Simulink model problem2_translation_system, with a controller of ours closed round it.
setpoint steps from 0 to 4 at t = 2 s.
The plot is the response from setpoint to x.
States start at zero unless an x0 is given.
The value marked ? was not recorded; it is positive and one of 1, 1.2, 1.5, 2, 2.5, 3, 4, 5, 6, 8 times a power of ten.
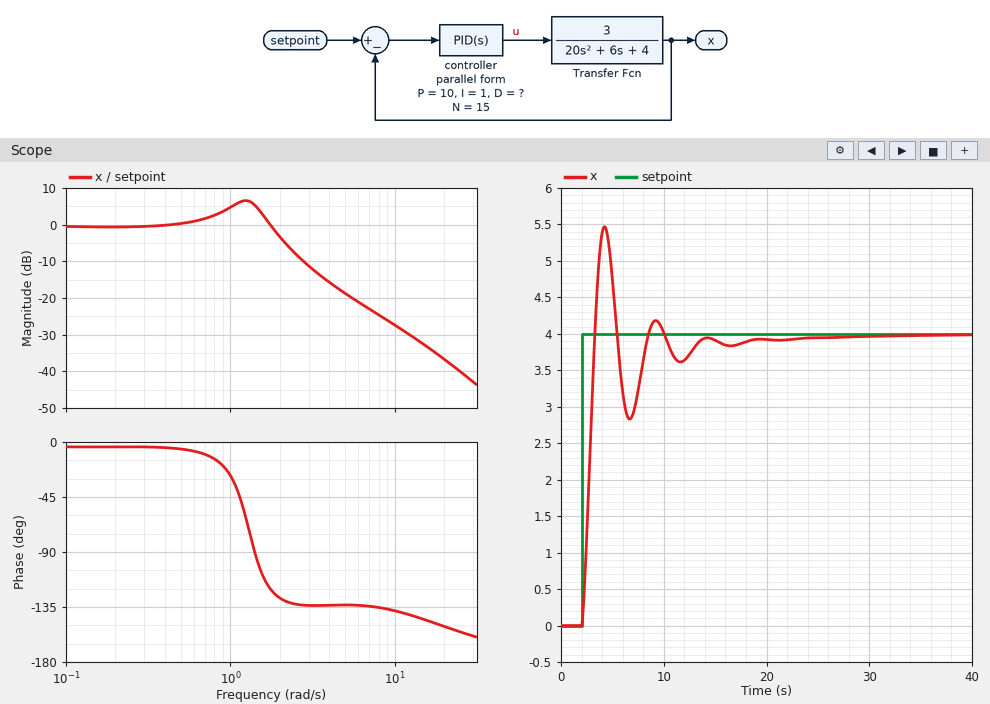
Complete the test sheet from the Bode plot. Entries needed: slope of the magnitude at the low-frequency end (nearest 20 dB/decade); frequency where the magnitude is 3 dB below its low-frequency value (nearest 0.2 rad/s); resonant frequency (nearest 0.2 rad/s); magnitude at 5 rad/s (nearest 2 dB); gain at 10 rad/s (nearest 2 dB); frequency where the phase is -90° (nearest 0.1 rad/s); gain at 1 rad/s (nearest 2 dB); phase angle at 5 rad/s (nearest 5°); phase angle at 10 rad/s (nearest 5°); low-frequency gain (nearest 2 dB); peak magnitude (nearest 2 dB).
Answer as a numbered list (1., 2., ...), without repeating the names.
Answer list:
1. 0 dB/decade
2. 2.0 rad/s
3. 1.2 rad/s
4. -18 dB
5. -28 dB
6. 1.4 rad/s
7. 4 dB
8. -135°
9. -140°
10. 0 dB
11. 6 dB
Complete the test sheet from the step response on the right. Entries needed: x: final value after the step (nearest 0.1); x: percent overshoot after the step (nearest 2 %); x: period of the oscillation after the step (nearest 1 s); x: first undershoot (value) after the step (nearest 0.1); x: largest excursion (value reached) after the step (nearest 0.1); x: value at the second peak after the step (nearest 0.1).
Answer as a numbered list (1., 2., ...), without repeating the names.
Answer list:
1. 4.0
2. 36 %
3. 5 s
4. 2.8
5. 5.5
6. 4.2
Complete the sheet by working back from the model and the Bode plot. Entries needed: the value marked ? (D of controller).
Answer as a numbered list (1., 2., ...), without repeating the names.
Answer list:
1. 2.5
